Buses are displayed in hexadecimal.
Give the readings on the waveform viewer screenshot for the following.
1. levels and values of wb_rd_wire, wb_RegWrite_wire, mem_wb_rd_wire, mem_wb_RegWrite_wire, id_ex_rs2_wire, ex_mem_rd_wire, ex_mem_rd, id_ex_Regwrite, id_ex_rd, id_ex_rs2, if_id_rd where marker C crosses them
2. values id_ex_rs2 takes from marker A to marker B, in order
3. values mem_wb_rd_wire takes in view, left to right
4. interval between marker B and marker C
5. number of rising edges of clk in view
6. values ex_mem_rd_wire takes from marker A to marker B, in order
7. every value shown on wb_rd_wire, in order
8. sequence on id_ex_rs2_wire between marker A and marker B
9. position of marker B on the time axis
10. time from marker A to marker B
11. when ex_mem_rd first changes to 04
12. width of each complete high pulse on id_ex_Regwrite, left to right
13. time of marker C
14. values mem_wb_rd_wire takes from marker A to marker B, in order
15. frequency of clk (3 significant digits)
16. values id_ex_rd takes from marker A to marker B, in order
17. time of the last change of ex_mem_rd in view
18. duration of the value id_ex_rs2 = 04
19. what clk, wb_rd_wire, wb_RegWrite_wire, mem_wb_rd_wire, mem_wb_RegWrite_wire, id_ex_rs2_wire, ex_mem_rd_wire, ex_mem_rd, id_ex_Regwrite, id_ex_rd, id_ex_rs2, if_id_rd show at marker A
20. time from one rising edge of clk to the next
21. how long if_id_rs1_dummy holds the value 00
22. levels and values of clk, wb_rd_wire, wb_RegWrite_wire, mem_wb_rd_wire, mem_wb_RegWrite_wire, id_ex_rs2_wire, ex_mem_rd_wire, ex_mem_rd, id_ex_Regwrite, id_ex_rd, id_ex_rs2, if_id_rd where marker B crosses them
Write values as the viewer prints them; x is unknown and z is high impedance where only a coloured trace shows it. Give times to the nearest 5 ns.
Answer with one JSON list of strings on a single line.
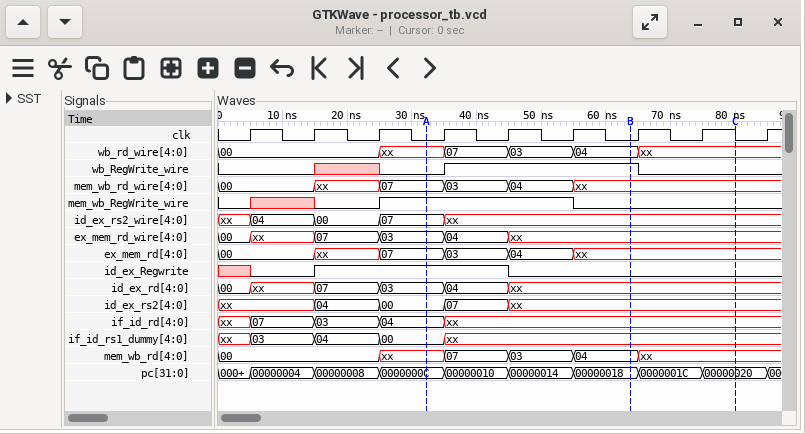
["wb_rd_wire=xx, wb_RegWrite_wire=0, mem_wb_rd_wire=xx, mem_wb_RegWrite_wire=0, id_ex_rs2_wire=xx, ex_mem_rd_wire=xx, ex_mem_rd=xx, id_ex_Regwrite=0, id_ex_rd=xx, id_ex_rs2=xx, if_id_rd=xx", "00, 07, xx", "00, xx, 07, 03, 04, xx", "15 ns", "9", "03, 04, xx", "00, xx, 07, 03, 04, xx", "07, xx", "65 ns", "30 ns", "45 ns", "30 ns", "80 ns", "07, 03, 04, xx", "100 MHz", "03, 04, xx", "55 ns", "10 ns", "clk=0, wb_rd_wire=xx, wb_RegWrite_wire=0, mem_wb_rd_wire=07, mem_wb_RegWrite_wire=1, id_ex_rs2_wire=07, ex_mem_rd_wire=03, ex_mem_rd=07, id_ex_Regwrite=1, id_ex_rd=03, id_ex_rs2=00, if_id_rd=04", "10 ns", "10 ns", "clk=0, wb_rd_wire=04, wb_RegWrite_wire=1, mem_wb_rd_wire=xx, mem_wb_RegWrite_wire=0, id_ex_rs2_wire=xx, ex_mem_rd_wire=xx, ex_mem_rd=xx, id_ex_Regwrite=0, id_ex_rd=xx, id_ex_rs2=xx, if_id_rd=xx"]
